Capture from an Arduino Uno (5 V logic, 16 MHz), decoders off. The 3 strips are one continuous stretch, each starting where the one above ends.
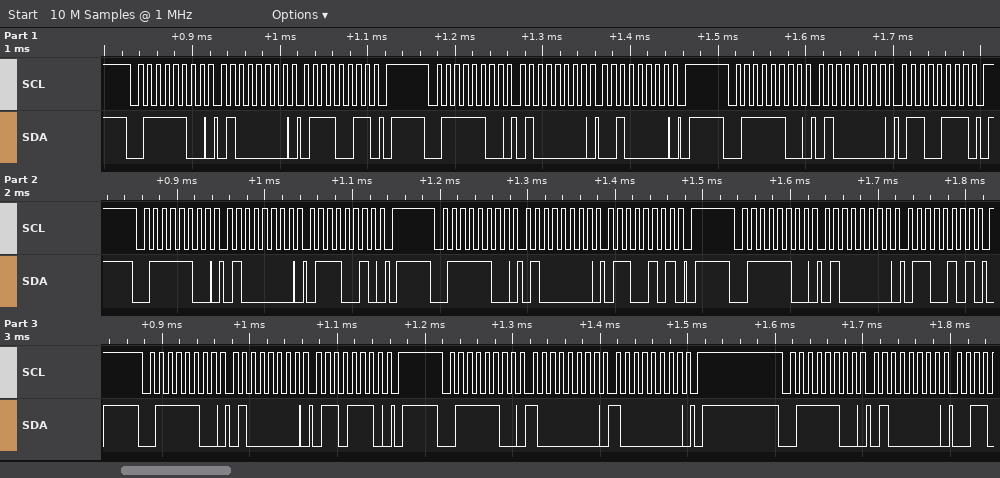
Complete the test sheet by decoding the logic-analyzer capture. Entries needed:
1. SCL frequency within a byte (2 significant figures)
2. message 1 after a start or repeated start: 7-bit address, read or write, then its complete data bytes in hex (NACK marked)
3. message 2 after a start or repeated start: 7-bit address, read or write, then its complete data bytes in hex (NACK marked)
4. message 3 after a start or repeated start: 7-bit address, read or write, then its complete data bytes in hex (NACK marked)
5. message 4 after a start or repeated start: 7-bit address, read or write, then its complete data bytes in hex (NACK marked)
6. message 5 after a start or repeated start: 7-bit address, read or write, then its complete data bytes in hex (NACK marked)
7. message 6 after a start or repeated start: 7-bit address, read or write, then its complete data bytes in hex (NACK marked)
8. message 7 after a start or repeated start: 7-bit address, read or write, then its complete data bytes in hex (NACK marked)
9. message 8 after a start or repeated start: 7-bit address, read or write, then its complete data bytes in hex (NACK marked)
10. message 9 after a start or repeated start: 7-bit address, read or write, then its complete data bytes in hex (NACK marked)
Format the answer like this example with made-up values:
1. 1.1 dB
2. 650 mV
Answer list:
1. 100 kHz
2. 0x3E write: 40 73
3. 0x3E write: 40 20
4. 0x3E write: 40 67
5. 0x3E write: 40 72
6. 0x3E write: 40 65
7. 0x3E write: 40 65
8. 0x3E write: 40 6E
9. 0x3E write: 80 80
10. 0x3E write: 40
